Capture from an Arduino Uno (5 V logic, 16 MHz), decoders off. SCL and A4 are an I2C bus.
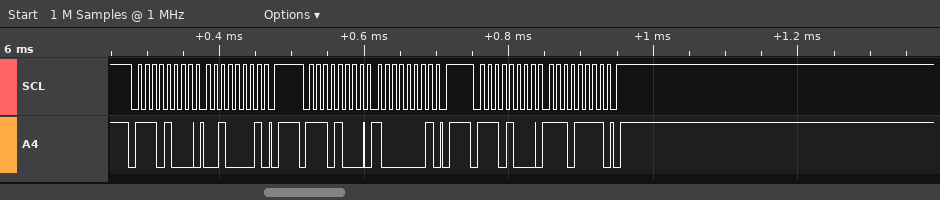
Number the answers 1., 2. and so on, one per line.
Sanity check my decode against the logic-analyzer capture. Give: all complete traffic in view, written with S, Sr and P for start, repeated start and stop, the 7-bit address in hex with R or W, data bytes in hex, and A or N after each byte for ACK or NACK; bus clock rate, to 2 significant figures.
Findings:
1. S 74W A 21 A P S 74W A 81 A P S 74W A EF A P
2. 100 kHz
